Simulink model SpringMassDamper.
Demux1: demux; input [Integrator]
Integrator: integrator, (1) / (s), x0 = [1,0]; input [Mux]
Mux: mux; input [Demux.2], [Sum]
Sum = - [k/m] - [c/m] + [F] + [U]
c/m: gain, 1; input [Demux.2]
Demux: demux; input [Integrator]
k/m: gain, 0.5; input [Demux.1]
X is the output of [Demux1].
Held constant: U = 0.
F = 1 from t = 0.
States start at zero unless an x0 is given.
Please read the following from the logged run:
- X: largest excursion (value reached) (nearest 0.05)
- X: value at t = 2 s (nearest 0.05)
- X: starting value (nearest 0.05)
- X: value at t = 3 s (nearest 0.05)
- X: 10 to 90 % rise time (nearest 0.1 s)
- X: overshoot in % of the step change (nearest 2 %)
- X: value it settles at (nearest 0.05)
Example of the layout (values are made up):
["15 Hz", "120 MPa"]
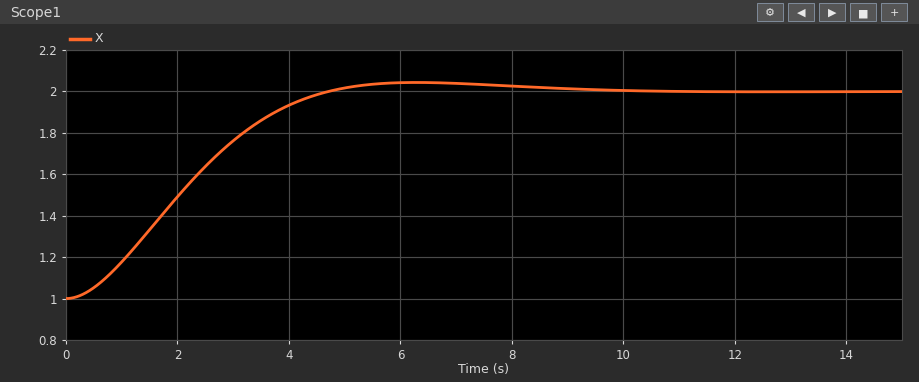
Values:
["2.05", "1.50", "1.00", "1.75", "3.0 s", "4 %", "2.00"]
